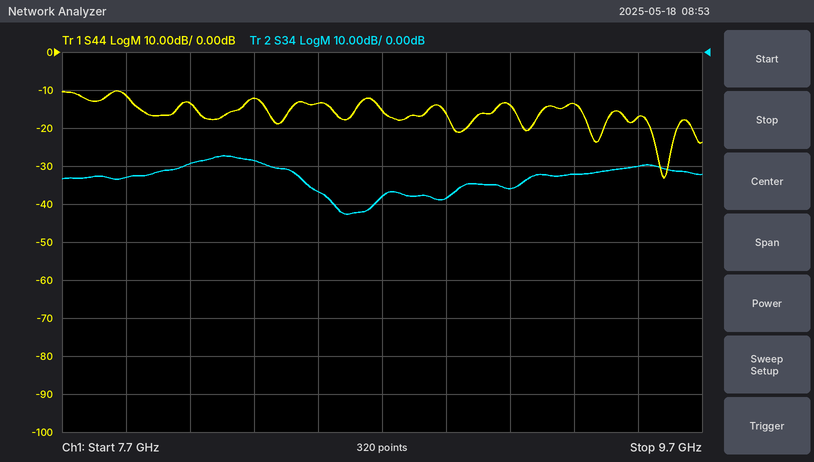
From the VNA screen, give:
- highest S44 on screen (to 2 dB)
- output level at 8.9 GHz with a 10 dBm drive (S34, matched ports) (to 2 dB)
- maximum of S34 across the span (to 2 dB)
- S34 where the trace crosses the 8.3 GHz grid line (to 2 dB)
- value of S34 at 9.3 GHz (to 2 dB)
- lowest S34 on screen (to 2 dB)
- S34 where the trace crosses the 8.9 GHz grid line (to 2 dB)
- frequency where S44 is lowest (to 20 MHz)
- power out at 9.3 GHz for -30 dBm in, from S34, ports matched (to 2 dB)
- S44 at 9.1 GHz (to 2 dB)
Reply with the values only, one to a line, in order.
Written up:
-10 dB
-28 dBm
-28 dB
-28 dB
-32 dB
-42 dB
-38 dB
9.58 GHz
-62 dBm
-14 dB
